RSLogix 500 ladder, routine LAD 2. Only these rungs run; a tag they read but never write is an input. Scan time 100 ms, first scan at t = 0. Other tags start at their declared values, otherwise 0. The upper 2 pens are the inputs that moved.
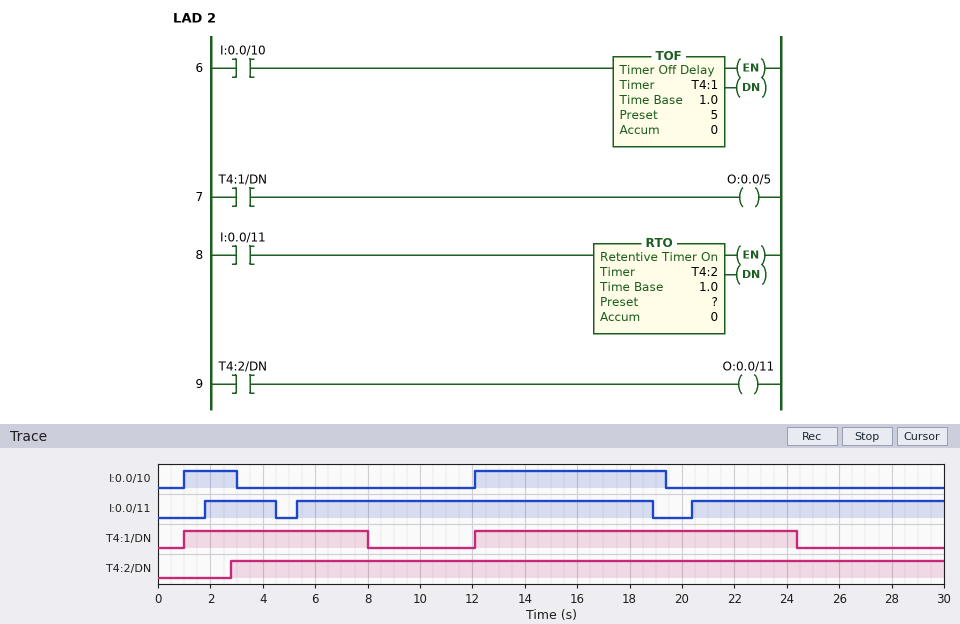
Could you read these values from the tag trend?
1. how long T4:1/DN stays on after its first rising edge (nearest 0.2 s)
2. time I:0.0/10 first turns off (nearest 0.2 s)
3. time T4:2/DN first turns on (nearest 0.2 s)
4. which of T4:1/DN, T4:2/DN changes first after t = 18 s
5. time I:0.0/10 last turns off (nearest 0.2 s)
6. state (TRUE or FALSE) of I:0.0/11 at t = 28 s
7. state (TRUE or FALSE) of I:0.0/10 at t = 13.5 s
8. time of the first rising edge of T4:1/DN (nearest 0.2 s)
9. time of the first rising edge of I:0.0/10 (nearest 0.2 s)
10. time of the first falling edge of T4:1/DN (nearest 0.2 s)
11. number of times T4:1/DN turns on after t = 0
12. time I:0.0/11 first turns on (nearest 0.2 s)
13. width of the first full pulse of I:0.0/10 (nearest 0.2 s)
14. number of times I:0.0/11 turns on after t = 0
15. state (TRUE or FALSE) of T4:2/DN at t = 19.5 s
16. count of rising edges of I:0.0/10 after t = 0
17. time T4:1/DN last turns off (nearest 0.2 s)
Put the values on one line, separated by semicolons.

7.0 s; 3.0 s; 2.8 s; T4:1/DN; 19.4 s; TRUE; TRUE; 1.0 s; 1.0 s; 8.0 s; 2; 1.8 s; 2.0 s; 3; TRUE; 2; 24.4 s
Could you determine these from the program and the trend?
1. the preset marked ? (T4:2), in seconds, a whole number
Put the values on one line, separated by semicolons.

1 s
